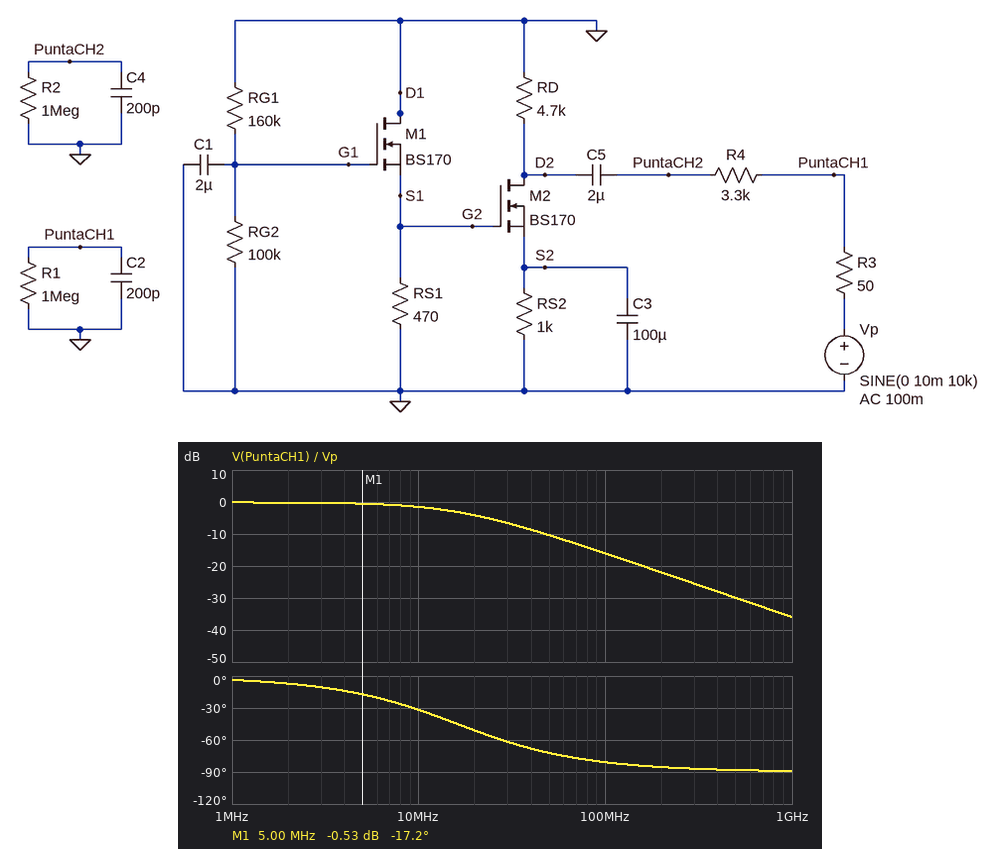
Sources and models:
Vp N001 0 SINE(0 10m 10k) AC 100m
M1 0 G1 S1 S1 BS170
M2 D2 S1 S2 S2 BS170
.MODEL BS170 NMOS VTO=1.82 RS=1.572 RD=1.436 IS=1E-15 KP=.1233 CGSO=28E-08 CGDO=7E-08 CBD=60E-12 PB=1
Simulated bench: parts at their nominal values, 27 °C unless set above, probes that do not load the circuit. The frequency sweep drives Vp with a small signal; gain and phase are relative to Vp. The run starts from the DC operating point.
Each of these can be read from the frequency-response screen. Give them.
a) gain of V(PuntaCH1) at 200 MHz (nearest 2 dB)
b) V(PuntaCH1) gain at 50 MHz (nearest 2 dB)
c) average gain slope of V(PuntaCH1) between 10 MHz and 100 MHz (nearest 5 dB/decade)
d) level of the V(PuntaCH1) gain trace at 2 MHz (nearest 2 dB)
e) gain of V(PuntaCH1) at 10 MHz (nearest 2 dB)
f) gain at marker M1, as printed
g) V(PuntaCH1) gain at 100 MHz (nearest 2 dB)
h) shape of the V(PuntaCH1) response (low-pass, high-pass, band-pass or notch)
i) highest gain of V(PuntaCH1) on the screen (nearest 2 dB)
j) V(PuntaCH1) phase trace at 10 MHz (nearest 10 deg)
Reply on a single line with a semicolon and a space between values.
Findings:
-22 dB; -10 dB; -15 dB/decade; 0 dB; -2 dB; -0.53 dB; -16 dB; low-pass; 0 dB; -30 deg
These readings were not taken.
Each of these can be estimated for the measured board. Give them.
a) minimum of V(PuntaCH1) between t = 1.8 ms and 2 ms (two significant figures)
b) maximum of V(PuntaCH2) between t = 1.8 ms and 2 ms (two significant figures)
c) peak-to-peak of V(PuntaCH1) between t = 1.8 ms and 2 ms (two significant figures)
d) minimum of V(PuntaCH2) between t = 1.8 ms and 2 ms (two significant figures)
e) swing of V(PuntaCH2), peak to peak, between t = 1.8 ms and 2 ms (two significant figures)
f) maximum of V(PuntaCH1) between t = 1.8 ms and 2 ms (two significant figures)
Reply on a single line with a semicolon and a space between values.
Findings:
-9.9 mV; 5.8 mV; 20 mV; -5.8 mV; 12 mV; 9.9 mV
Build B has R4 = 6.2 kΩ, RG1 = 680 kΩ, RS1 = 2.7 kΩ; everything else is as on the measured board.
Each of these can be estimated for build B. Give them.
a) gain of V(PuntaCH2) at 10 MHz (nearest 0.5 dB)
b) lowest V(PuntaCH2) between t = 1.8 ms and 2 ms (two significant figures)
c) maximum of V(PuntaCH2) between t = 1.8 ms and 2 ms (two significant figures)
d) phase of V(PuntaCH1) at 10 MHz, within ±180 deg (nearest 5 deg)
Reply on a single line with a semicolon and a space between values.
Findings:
-42.0 dB; -4.3 mV; 4.3 mV; -30 deg
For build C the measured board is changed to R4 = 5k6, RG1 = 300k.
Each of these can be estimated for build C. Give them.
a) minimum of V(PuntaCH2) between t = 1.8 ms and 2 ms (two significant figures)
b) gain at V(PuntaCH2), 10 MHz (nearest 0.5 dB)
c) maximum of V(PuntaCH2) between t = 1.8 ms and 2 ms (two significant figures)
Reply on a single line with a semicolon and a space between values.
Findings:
-4.5 mV; -41.0 dB; 4.5 mV
